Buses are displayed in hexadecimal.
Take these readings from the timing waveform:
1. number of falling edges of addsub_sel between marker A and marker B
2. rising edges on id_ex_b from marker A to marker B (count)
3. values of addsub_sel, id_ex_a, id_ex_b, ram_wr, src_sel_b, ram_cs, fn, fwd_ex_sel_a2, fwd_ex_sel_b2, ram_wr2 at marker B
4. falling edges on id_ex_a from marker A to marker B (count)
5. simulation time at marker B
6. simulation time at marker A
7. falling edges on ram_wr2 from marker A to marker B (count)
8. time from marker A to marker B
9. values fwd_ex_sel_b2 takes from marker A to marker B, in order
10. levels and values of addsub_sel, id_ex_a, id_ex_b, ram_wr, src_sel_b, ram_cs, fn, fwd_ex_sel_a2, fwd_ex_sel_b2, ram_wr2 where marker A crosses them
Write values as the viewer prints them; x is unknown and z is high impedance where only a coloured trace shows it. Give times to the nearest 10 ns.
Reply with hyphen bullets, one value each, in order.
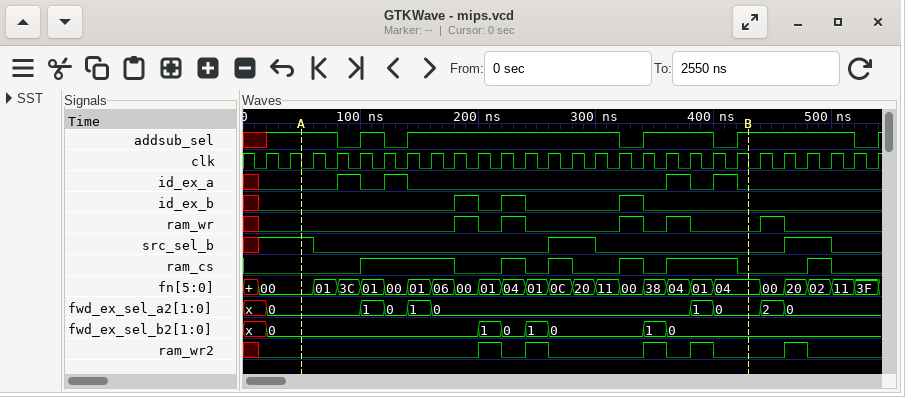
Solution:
- 4
- 3
- addsub_sel=1, id_ex_a=0, id_ex_b=0, ram_wr=0, src_sel_b=0, ram_cs=0, fn=04, fwd_ex_sel_a2=0, fwd_ex_sel_b2=0, ram_wr2=0
- 4
- 430 ns
- 50 ns
- 4
- 380 ns
- 0, 1, 0, 1, 0, 1, 0
- addsub_sel=1, id_ex_a=0, id_ex_b=0, ram_wr=0, src_sel_b=1, ram_cs=0, fn=00, fwd_ex_sel_a2=0, fwd_ex_sel_b2=0, ram_wr2=0
